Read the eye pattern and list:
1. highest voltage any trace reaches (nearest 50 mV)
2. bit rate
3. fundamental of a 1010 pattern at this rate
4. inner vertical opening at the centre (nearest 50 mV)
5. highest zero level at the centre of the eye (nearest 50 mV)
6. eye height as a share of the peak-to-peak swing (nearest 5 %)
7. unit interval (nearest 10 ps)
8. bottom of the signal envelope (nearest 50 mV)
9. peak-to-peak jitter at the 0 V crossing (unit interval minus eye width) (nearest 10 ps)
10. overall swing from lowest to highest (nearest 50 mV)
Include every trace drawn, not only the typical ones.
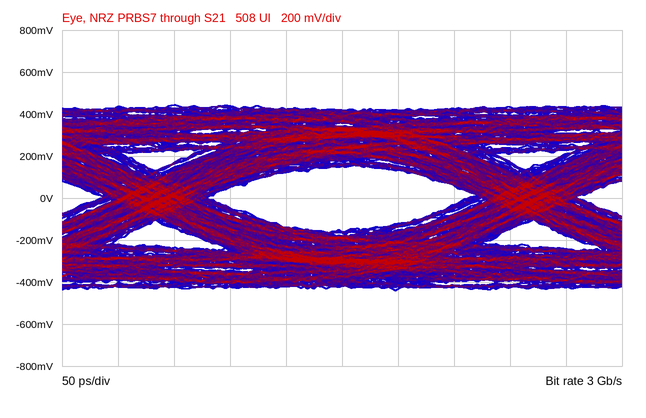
450 mV
3 Gb/s
1.5 GHz
300 mV
-150 mV
35 %
330 ps
-450 mV
100 ps
900 mV
